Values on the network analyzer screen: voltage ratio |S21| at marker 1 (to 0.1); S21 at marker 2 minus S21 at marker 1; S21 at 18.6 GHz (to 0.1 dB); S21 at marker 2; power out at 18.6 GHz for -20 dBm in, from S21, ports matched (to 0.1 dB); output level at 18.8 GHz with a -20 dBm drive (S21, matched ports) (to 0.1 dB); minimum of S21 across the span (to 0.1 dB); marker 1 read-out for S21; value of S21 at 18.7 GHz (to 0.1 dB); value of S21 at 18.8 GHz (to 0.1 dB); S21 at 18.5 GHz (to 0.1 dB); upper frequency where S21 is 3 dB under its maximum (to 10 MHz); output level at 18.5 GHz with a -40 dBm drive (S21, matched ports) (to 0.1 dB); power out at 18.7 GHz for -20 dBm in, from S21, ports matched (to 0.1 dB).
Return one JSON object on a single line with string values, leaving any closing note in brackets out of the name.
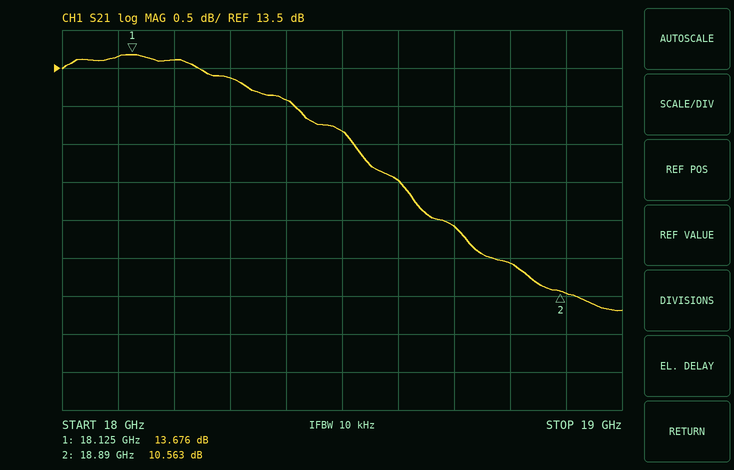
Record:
{"voltage ratio |S21| at marker 1": "4.8", "S21 at marker 2 minus S21 at marker 1": "-3.113 dB", "S21 at 18.6 GHz": "12.0 dB", "S21 at marker 2": "10.563 dB", "power out at 18.6 GHz for -20 dBm in, from S21, ports matched": "-8.0 dBm", "output level at 18.8 GHz with a -20 dBm drive (S21, matched ports)": "-9.1 dBm", "minimum of S21 across the span": "10.3 dB", "marker 1 read-out for S21": "13.676 dB", "value of S21 at 18.7 GHz": "11.4 dB", "value of S21 at 18.8 GHz": "10.9 dB", "S21 at 18.5 GHz": "12.7 dB", "upper frequency where S21 is 3 dB under its maximum": "18.85 GHz", "output level at 18.5 GHz with a -40 dBm drive (S21, matched ports)": "-27.3 dBm", "power out at 18.7 GHz for -20 dBm in, from S21, ports matched": "-8.6 dBm"}
